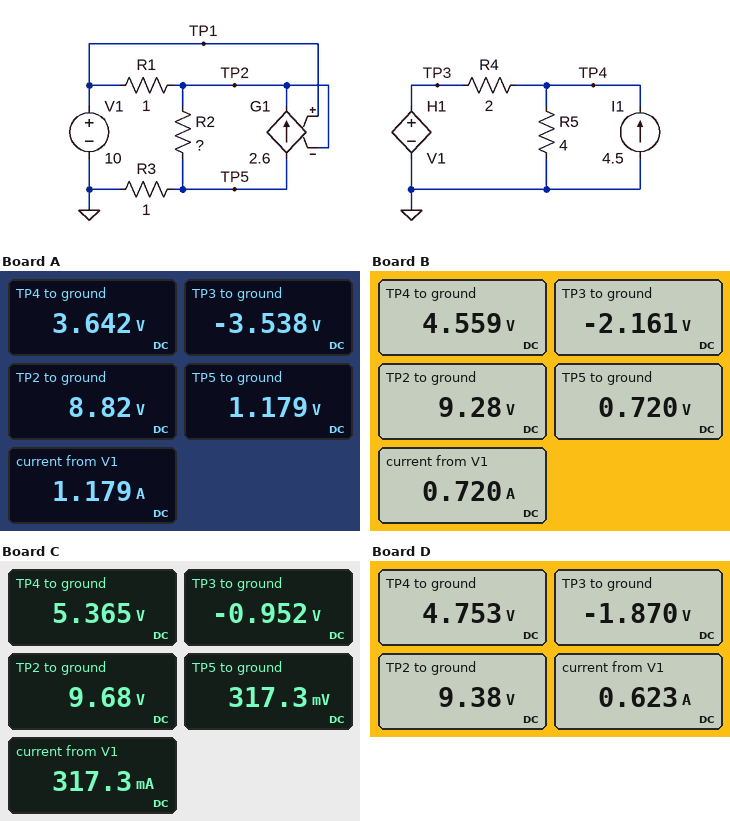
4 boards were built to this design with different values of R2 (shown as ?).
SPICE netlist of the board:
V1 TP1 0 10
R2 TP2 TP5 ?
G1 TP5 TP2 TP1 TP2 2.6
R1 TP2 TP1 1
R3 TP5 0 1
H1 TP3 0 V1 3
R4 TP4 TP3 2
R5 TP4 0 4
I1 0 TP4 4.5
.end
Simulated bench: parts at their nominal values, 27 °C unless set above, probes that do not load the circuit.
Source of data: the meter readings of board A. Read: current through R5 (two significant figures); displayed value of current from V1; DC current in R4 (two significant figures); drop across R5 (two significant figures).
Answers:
910 mA
1.179 A
3.6 A
3.6 V
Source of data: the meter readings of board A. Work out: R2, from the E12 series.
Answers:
1.8 Ω
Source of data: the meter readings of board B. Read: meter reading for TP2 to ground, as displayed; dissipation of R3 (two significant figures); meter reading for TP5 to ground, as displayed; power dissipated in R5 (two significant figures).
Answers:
9.28 V
520 mW
0.720 V
5.2 W
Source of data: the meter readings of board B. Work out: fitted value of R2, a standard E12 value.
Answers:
3.3 Ω
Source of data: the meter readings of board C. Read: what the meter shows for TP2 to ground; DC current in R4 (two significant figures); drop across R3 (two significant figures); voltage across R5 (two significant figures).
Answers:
9.68 V
3.2 A
320 mV
5.4 V
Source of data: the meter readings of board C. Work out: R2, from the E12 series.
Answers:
8.2 Ω
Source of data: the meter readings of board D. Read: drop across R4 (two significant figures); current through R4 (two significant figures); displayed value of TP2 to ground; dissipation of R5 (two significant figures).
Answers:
6.6 V
3.3 A
9.38 V
5.6 W
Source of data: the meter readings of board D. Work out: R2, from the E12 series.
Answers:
3.9 Ω
